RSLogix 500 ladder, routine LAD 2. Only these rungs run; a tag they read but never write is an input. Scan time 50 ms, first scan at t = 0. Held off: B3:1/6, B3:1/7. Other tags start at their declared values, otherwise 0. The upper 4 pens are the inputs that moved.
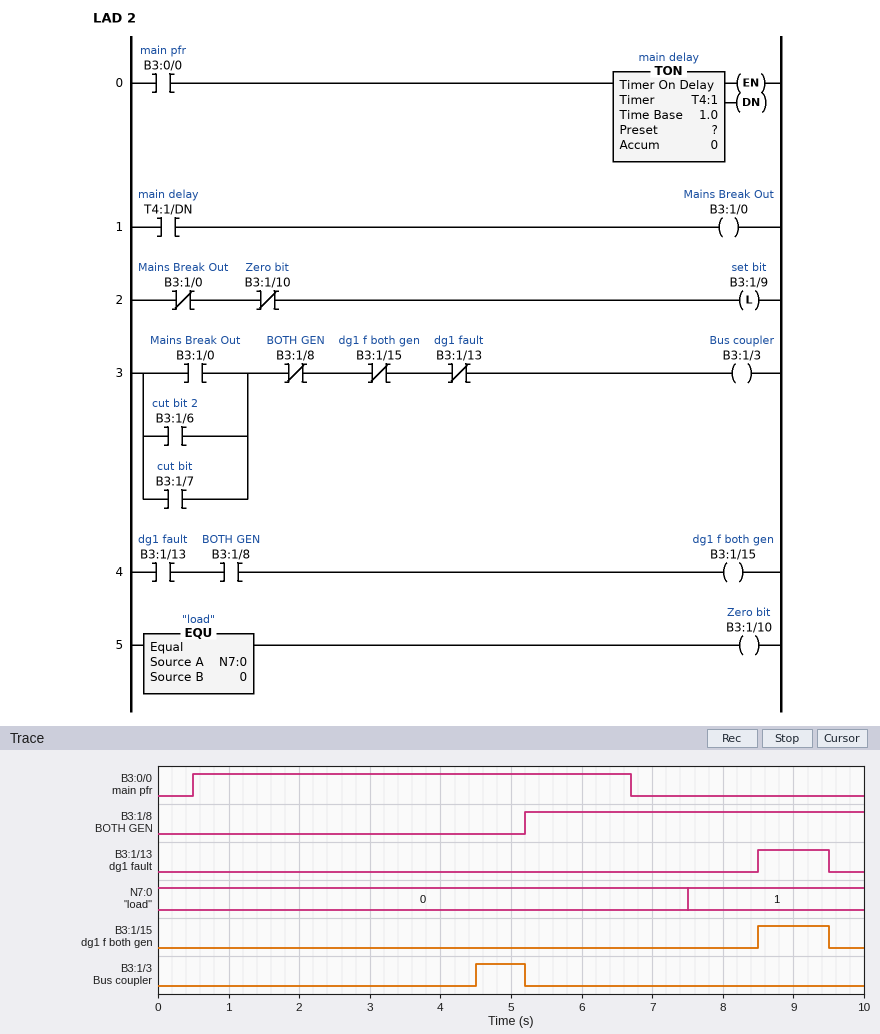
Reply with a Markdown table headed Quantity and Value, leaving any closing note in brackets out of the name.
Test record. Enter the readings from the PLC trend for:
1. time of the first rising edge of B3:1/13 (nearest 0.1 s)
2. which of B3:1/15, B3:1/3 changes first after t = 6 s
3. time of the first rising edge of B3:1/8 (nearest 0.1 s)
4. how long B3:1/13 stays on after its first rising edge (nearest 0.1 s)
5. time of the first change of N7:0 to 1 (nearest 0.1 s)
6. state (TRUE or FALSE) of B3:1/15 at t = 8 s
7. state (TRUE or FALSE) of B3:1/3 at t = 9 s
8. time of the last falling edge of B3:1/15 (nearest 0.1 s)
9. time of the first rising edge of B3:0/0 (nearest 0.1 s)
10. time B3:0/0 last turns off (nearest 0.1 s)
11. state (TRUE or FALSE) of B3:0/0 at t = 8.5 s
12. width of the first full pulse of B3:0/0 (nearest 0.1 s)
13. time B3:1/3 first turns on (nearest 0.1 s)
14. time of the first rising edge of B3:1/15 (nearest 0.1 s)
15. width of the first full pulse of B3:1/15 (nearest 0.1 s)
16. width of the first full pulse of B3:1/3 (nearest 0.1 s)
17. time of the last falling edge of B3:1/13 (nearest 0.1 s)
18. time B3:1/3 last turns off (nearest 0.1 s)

| Quantity | Value |
|---|---|
| time of the first rising edge of B3:1/13 | 8.5 s |
| which of B3:1/15, B3:1/3 changes first after t = 6 s | B3:1/15 |
| time of the first rising edge of B3:1/8 | 5.2 s |
| how long B3:1/13 stays on after its first rising edge | 1.0 s |
| time of the first change of N7:0 to 1 | 7.5 s |
| state (TRUE or FALSE) of B3:1/15 at t = 8 s | FALSE |
| state (TRUE or FALSE) of B3:1/3 at t = 9 s | FALSE |
| time of the last falling edge of B3:1/15 | 9.5 s |
| time of the first rising edge of B3:0/0 | 0.5 s |
| time B3:0/0 last turns off | 6.7 s |
| state (TRUE or FALSE) of B3:0/0 at t = 8.5 s | FALSE |
| width of the first full pulse of B3:0/0 | 6.2 s |
| time B3:1/3 first turns on | 4.5 s |
| time of the first rising edge of B3:1/15 | 8.5 s |
| width of the first full pulse of B3:1/15 | 1.0 s |
| width of the first full pulse of B3:1/3 | 0.7 s |
| time of the last falling edge of B3:1/13 | 9.5 s |
| time B3:1/3 last turns off | 5.2 s |
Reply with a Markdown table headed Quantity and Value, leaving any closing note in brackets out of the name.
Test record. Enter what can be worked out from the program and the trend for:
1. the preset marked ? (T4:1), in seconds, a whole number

| Quantity | Value |
|---|---|
| the preset marked ? (T4:1), in seconds, a whole number | 4 s |
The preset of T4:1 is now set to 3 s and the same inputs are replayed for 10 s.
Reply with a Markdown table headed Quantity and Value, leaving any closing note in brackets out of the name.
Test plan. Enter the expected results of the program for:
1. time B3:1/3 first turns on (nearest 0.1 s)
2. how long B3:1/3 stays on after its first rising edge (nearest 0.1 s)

| Quantity | Value |
|---|---|
| time B3:1/3 first turns on | 3.5 s |
| how long B3:1/3 stays on after its first rising edge | 1.7 s |
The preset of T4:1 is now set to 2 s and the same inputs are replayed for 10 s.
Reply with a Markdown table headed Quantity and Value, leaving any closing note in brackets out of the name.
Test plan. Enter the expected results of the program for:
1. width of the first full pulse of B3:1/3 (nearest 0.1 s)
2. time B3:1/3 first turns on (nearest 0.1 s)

| Quantity | Value |
|---|---|
| width of the first full pulse of B3:1/3 | 2.7 s |
| time B3:1/3 first turns on | 2.5 s |
